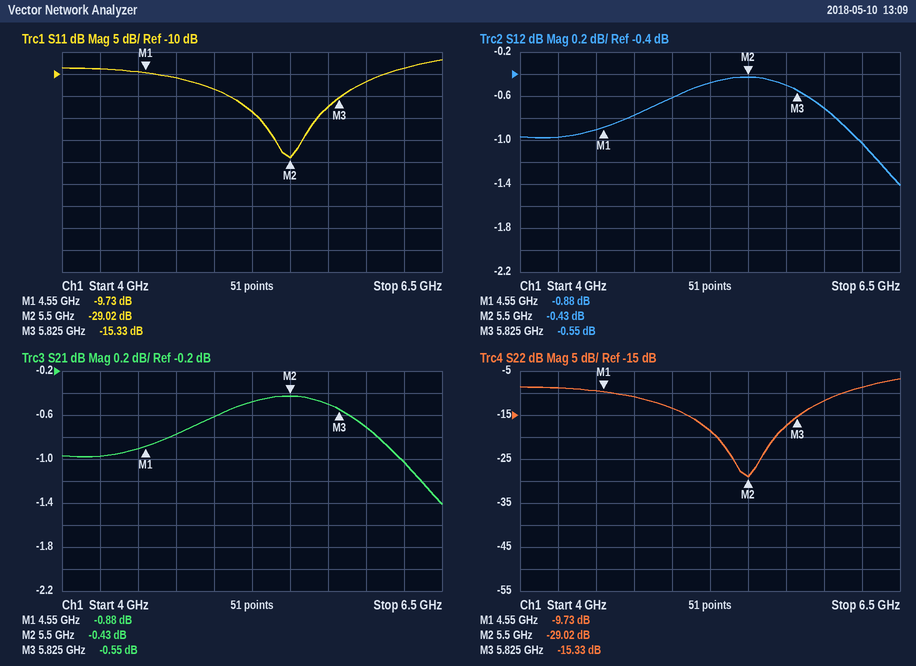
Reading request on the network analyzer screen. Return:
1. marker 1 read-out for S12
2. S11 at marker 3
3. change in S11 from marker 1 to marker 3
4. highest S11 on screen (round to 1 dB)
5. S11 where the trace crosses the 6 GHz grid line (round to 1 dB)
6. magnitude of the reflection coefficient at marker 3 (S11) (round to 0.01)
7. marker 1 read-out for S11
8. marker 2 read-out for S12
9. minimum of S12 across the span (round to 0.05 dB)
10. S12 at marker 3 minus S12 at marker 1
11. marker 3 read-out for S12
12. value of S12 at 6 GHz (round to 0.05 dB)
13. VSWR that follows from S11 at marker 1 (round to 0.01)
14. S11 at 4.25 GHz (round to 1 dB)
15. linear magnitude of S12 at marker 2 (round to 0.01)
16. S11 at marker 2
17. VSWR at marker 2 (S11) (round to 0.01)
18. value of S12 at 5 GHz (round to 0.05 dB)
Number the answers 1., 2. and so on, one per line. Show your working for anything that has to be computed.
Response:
1. -0.88 dB
2. -15.33 dB
3. -15.33 − (-9.73) = -5.60 dB
4. -7 dB
5. -12 dB
6. 10^(-15.33/20) ≈ 0.17
7. -9.73 dB
8. -0.43 dB
9. -1.40 dB
10. -0.55 − (-0.88) = 0.33 dB
11. -0.55 dB
12. -0.70 dB
13. (1 + 0.3262)/(1 − 0.3262) ≈ 1.97
14. -9 dB
15. 10^(-0.43/20) ≈ 0.95
16. -29.02 dB
17. (1 + 0.0354)/(1 − 0.0354) ≈ 1.07
18. -0.60 dB
